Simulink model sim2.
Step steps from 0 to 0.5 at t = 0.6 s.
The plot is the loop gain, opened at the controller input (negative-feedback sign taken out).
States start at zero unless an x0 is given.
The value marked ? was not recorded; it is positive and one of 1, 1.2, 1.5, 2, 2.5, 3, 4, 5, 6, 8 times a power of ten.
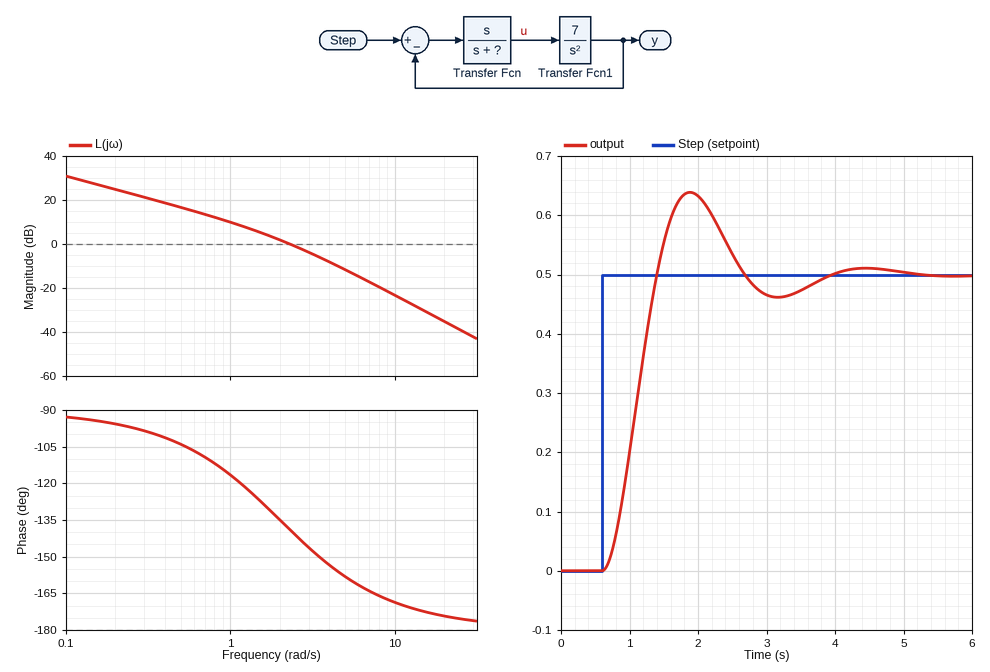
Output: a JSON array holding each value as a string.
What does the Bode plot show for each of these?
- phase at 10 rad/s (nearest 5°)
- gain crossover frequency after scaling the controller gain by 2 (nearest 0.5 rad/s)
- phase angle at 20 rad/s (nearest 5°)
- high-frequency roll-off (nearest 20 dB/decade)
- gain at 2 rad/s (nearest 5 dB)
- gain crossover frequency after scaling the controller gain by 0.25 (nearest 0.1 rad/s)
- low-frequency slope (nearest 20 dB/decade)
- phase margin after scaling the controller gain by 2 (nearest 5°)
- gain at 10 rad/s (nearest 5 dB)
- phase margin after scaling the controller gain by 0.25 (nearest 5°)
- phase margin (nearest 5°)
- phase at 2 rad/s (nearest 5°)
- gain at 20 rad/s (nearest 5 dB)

["-170°", "3.5 rad/s", "-175°", "-40 dB/decade", "0 dB", "0.8 rad/s", "-20 dB/decade", "30°", "-25 dB", "70°", "40°", "-135°", "-35 dB"]
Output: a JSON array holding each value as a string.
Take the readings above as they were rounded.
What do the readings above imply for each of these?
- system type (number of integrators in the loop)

["1"]
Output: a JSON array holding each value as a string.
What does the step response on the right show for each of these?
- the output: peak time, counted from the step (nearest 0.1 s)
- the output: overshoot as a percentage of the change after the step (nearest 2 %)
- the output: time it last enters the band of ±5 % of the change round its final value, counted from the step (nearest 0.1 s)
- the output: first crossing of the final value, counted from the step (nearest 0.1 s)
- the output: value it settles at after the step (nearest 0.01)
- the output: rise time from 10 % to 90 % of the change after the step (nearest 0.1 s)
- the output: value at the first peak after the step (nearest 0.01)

["1.3 s", "28 %", "2.9 s", "0.8 s", "0.50", "0.5 s", "0.64"]
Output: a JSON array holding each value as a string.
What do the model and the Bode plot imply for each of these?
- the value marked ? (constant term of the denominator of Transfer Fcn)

["2"]
